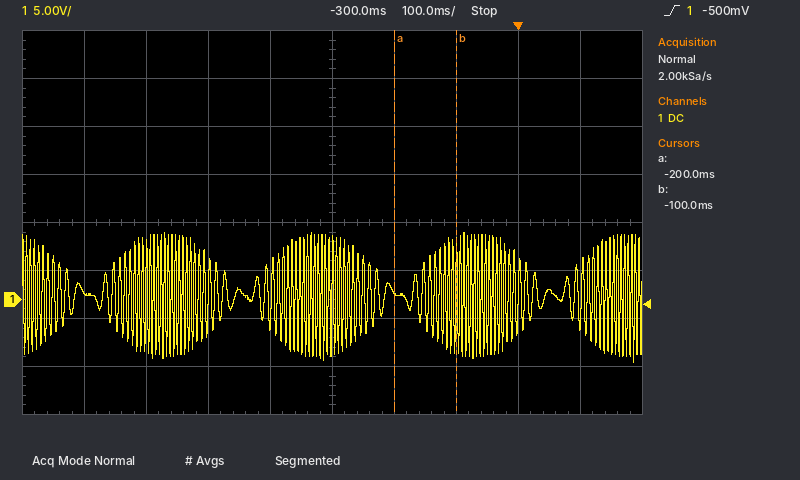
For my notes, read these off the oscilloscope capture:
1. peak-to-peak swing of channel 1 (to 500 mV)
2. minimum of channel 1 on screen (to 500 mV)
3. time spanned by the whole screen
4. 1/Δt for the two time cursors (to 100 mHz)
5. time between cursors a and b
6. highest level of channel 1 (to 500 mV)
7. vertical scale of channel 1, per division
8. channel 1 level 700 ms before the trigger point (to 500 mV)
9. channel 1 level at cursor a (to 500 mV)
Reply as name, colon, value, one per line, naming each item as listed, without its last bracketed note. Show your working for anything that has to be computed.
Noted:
peak-to-peak swing of channel 1: 7.0 V − (-6.5 V) = 13.5 V
minimum of channel 1 on screen: -6.5 V
time spanned by the whole screen: 1 s
1/Δt for the two time cursors: 1 / 100 ms ≈ 10.0 Hz
time between cursors a and b: -100 ms − (-200 ms) = 100 ms
highest level of channel 1: 7.0 V
vertical scale of channel 1, per division: 5 V
channel 1 level 700 ms before the trigger point: 1.0 V
channel 1 level at cursor a: 1.0 V
